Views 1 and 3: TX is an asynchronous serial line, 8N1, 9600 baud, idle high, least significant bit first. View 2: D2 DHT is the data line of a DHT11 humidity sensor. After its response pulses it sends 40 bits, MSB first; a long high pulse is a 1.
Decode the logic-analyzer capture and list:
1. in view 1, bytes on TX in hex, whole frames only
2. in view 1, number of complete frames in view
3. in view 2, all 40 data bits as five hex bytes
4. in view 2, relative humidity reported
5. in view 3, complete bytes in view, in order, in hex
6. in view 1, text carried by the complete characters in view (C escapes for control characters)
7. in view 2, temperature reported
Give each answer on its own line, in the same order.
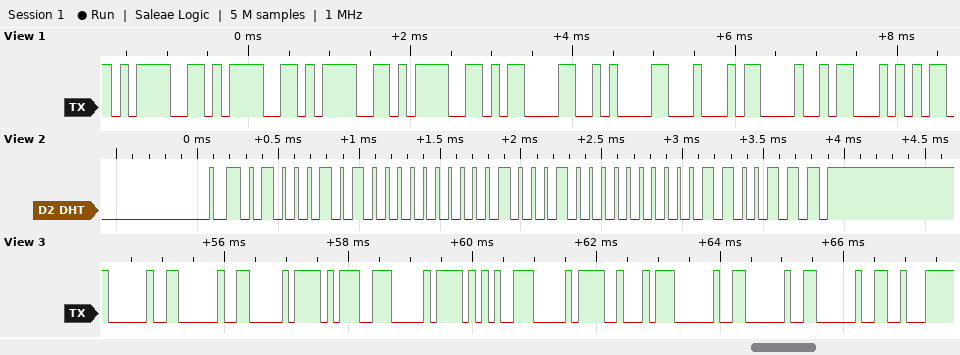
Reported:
3D 3D 3D 3D 0D 0A 44 48 54
9
45 00 22 00 67
69 %
20 20 D0 9D D0 95 D0 A2 20 20 20 E2
"====\r\nDHT"
34.0 °C
